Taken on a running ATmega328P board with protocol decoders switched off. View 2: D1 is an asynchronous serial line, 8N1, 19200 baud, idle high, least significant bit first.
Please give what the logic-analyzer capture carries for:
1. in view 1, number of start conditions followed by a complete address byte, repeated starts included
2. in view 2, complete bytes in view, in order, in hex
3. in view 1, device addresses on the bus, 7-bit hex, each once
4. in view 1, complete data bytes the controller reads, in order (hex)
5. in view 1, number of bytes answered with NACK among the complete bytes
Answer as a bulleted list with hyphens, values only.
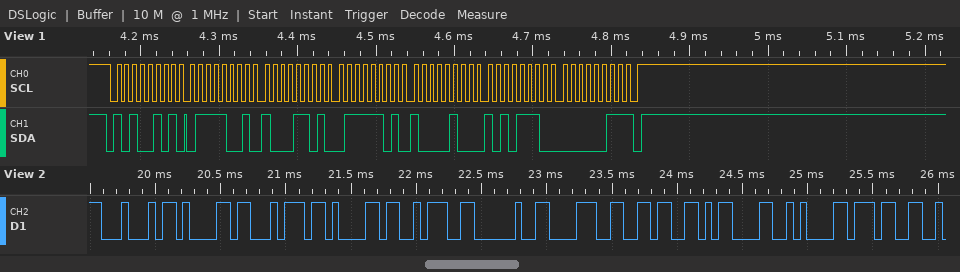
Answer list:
- 1
- 44 61 74 61 3A 20 38 36 0D 0A 37
- 0x52
- 79 8D 7D 84 AE 03
- 1
